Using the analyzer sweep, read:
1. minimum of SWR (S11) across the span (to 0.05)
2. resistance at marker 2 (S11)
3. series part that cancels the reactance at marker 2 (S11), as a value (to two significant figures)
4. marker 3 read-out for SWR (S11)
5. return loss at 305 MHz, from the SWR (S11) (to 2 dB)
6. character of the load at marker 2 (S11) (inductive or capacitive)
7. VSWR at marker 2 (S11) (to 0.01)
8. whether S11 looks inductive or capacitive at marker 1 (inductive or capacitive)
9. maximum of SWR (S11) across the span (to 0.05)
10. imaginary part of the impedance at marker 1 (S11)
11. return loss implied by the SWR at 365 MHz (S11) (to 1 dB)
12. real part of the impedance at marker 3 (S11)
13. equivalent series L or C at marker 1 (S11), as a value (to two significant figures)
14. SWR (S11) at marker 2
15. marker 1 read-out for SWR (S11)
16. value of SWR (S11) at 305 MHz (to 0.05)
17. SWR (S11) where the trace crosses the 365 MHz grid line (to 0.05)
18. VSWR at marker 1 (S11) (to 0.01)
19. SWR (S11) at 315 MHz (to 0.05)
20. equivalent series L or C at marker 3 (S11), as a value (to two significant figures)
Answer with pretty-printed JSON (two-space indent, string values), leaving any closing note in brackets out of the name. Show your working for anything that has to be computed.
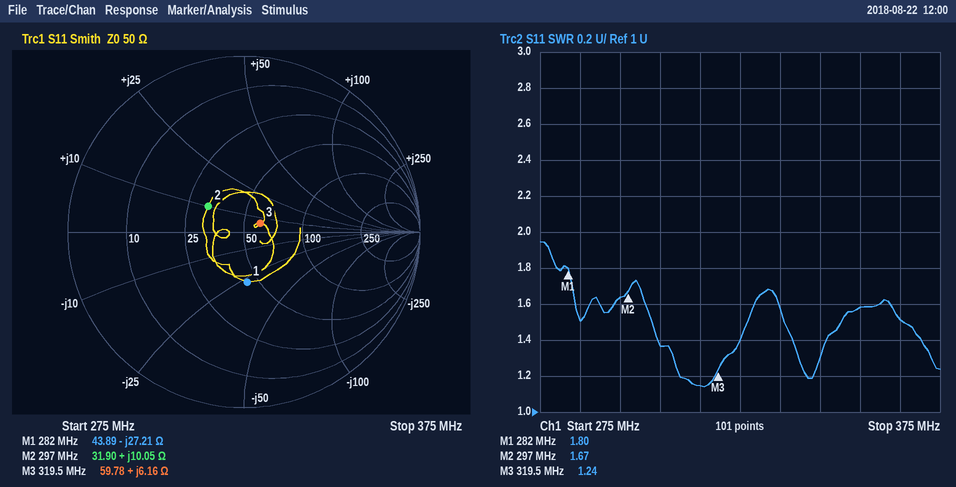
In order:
{
  "minimum of SWR (S11) across the span": "1.15",
  "resistance at marker 2": "31.90 Ω",
  "series part that cancels the reactance at marker 2 (S11), as a value": "C = 1/(2π × 297 MHz × 10.05 Ω) ≈ 53 pF",
  "marker 3 read-out for SWR": "1.24",
  "return loss at 305 MHz, from the SWR (S11)": "−20 log10((1.35 − 1)/(1.35 + 1)) ≈ 16 dB",
  "character of the load at marker 2 (S11)": "inductive",
  "VSWR at marker 2 (S11)": "1.67",
  "whether S11 looks inductive or capacitive at marker 1": "capacitive",
  "maximum of SWR (S11) across the span": "1.95",
  "imaginary part of the impedance at marker 1": "-27.21 Ω",
  "return loss implied by the SWR at 365 MHz (S11)": "−20 log10((1.5 − 1)/(1.5 + 1)) ≈ 14 dB",
  "real part of the impedance at marker 3": "59.78 Ω",
  "equivalent series L or C at marker 1 (S11), as a value": "C = 1/(2π × 282 MHz × 27.21 Ω) ≈ 21 pF",
  "SWR (S11) at marker 2": "1.67",
  "marker 1 read-out for SWR": "1.80",
  "value of SWR (S11) at 305 MHz": "1.35",
  "SWR (S11) where the trace crosses the 365 MHz grid line": "1.50",
  "VSWR at marker 1 (S11)": "1.80",
  "SWR (S11) at 315 MHz": "1.15",
  "equivalent series L or C at marker 3 (S11), as a value": "L = 6.16 Ω/(2π × 319.5 MHz) ≈ 3.1 nH"
}
